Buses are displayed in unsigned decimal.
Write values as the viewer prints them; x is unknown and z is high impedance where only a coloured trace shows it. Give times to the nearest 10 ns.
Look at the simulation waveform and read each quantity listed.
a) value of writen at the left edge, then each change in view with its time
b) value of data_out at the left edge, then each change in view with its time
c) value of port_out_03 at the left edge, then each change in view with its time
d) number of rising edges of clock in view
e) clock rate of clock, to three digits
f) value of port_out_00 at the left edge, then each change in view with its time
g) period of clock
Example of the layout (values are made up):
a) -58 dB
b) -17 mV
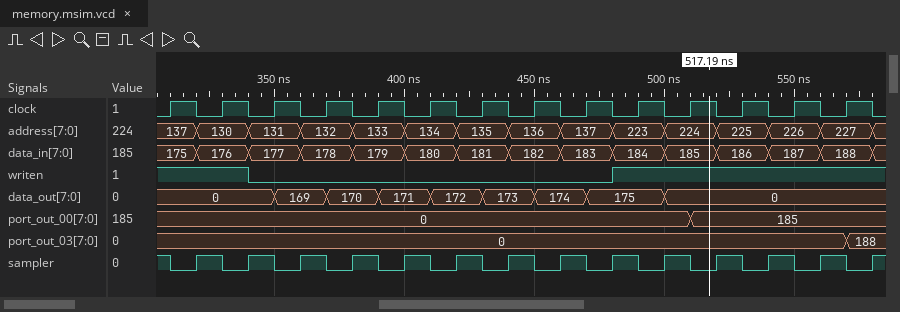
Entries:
a) 1, 0 at 340 ns, 1 at 480 ns
b) 0, 169 at 350 ns, 170 at 370 ns, 171 at 390 ns, 172 at 410 ns, 173 at 430 ns, 174 at 450 ns, 175 at 470 ns, 0 at 500 ns
c) 0, 188 at 570 ns
d) 14
e) 50.0 MHz
f) 0, 185 at 510 ns
g) 20 ns
